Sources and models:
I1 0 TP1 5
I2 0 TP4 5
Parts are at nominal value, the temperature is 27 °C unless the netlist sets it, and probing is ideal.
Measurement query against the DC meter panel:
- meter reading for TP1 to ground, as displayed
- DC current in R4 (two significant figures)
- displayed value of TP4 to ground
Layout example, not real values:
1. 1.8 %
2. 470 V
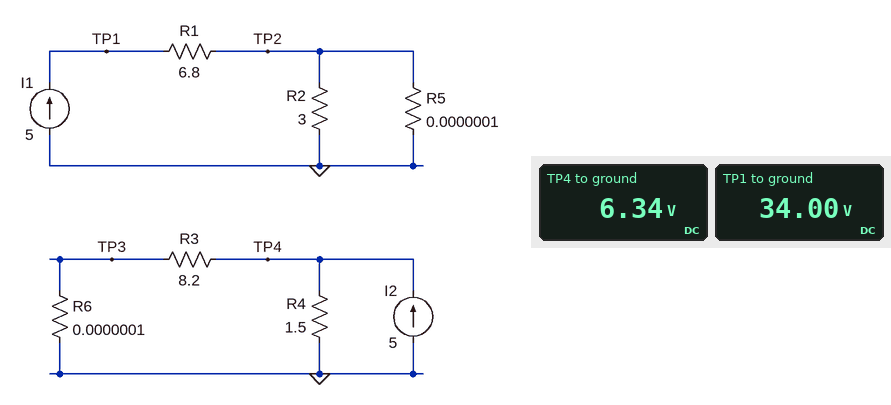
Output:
1. 34.00 V
2. 4.2 A
3. 6.34 V
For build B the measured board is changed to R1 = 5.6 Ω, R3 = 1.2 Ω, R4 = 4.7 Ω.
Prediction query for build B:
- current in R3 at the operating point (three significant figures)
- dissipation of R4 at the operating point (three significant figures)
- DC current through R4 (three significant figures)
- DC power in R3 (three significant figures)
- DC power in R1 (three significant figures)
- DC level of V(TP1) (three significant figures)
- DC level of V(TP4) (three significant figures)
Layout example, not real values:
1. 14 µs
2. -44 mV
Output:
1. 3.98 A
2. 4.86 W
3. 1.02 A
4. 19.0 W
5. 140 W
6. 28.0 V
7. 4.78 V
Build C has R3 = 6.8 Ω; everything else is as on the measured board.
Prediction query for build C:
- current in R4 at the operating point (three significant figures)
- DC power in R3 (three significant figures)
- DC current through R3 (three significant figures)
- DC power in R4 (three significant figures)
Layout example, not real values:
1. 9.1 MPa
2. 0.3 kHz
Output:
1. 4.10 A
2. 5.55 W
3. 904 mA
4. 25.2 W
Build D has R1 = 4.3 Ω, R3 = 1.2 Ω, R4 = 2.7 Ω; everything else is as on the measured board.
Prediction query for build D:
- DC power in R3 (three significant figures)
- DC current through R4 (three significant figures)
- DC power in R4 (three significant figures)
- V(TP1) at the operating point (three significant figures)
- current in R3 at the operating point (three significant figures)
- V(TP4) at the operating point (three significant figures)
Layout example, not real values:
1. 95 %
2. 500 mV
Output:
1. 14.4 W
2. 1.54 A
3. 6.39 W
4. 21.5 V
5. 3.46 A
6. 4.15 V
